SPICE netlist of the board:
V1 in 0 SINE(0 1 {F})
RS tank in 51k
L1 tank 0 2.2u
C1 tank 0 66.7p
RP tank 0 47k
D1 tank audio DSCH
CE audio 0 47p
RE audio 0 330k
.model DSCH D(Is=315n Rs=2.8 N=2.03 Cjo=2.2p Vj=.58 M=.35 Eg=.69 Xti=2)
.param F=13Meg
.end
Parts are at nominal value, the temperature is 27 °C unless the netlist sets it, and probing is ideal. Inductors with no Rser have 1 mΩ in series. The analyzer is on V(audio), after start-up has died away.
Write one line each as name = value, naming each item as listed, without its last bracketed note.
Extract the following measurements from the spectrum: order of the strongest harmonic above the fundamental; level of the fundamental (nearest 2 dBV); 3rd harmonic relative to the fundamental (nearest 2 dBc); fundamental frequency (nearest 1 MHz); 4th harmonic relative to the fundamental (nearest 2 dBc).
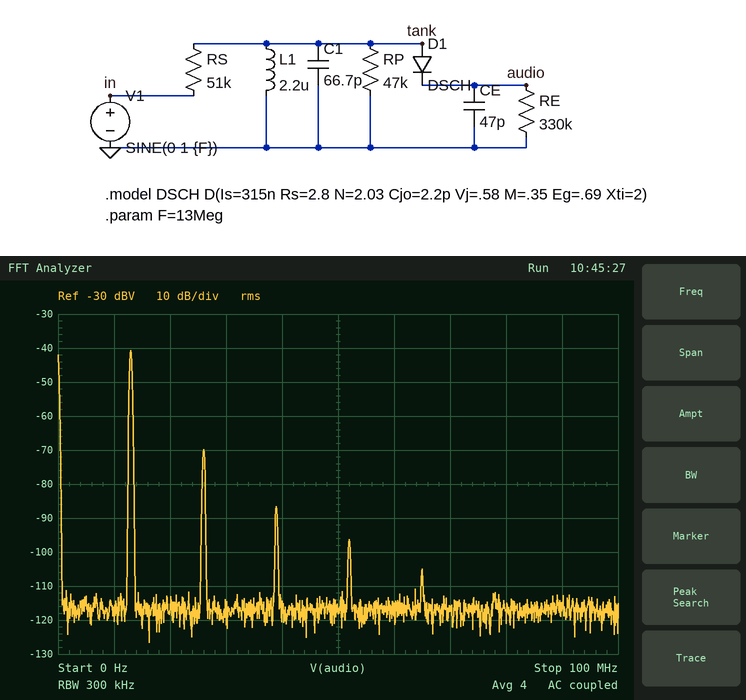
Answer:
order of the strongest harmonic above the fundamental = 2
level of the fundamental = -40 dBV
3rd harmonic relative to the fundamental = -46 dBc
fundamental frequency = 13 MHz
4th harmonic relative to the fundamental = -56 dBc
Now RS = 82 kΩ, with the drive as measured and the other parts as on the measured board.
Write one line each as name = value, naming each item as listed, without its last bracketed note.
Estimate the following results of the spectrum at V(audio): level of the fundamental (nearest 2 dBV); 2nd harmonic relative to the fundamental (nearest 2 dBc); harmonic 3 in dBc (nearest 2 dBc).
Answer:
level of the fundamental = -44 dBV
2nd harmonic relative to the fundamental = -32 dBc
harmonic 3 in dBc = -50 dBc
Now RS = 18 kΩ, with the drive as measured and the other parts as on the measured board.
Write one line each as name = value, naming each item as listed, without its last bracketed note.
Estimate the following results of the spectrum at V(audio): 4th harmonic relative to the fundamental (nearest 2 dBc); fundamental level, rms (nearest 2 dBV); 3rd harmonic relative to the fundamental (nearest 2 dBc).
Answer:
4th harmonic relative to the fundamental = -48 dBc
fundamental level, rms = -36 dBV
3rd harmonic relative to the fundamental = -40 dBc
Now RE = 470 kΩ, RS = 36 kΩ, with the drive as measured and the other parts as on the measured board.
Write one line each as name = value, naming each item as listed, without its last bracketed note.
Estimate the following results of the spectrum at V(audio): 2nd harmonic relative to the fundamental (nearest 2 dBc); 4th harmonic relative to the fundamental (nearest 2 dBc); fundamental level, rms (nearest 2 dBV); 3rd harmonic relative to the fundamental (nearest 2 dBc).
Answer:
2nd harmonic relative to the fundamental = -28 dBc
4th harmonic relative to the fundamental = -54 dBc
fundamental level, rms = -38 dBV
3rd harmonic relative to the fundamental = -44 dBc
